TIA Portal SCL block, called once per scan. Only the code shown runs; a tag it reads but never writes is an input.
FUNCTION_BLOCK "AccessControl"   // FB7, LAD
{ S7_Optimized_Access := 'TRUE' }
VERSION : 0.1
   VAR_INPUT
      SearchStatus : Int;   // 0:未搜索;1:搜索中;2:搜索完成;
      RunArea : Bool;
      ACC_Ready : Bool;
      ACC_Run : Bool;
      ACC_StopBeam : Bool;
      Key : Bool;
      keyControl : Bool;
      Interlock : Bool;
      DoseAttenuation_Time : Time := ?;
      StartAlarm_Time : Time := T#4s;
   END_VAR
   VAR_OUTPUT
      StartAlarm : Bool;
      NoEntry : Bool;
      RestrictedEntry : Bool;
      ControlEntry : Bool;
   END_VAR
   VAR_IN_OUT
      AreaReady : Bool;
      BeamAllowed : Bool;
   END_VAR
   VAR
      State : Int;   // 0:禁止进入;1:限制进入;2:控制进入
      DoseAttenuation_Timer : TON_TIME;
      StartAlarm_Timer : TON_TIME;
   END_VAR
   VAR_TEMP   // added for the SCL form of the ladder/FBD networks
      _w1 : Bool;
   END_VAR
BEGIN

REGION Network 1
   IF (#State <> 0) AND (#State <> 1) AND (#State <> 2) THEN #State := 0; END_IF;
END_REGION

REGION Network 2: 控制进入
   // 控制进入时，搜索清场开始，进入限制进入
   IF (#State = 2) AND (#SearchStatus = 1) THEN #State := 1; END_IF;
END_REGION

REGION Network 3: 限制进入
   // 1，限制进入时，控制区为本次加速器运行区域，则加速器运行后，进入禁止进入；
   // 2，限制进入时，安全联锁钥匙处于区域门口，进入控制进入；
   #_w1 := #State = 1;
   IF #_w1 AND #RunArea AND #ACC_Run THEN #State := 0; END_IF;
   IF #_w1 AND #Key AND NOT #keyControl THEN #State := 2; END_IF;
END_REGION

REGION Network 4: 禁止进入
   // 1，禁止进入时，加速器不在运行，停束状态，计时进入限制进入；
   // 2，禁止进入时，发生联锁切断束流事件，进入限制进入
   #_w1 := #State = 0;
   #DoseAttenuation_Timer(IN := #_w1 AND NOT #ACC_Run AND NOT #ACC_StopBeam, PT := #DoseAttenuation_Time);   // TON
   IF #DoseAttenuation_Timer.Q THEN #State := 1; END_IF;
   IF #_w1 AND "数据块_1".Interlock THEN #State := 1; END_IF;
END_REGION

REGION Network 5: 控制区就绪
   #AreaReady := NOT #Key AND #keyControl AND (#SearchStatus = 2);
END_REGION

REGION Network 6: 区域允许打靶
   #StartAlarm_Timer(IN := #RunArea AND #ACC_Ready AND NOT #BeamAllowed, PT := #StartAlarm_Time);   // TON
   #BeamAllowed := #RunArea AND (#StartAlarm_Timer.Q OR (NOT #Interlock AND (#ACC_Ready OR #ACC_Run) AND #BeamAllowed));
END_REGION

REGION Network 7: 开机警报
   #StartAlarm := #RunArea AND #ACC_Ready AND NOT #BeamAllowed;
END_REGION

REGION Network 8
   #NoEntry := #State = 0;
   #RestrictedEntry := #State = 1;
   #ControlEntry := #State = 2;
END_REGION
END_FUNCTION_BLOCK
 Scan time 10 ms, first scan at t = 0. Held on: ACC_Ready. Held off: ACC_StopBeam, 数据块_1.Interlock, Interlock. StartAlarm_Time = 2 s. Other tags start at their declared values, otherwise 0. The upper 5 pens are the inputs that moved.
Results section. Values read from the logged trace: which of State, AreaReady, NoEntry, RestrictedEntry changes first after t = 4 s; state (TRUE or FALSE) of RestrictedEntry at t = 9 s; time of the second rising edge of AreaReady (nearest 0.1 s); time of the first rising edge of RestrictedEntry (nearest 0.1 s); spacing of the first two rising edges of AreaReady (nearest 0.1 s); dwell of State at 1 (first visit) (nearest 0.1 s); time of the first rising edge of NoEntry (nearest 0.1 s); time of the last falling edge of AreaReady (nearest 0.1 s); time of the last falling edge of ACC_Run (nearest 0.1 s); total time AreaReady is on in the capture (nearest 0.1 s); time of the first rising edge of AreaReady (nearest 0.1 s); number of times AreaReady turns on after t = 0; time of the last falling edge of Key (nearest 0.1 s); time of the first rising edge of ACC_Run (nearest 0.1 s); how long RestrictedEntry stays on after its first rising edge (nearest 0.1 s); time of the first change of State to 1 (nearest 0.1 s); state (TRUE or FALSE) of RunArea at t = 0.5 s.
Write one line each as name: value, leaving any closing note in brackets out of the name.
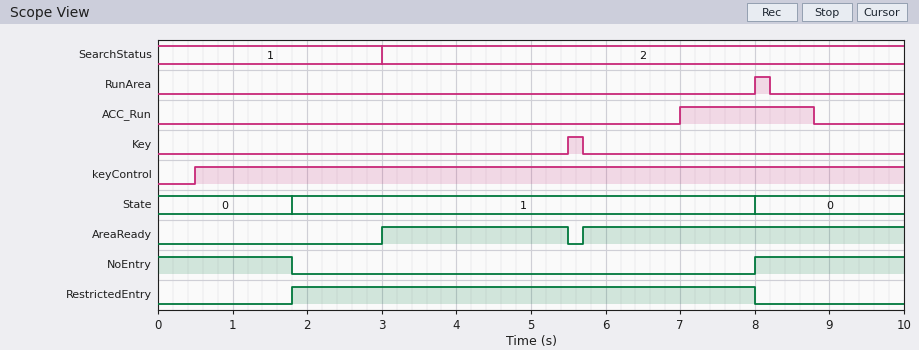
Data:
which of State, AreaReady, NoEntry, RestrictedEntry changes first after t = 4 s: AreaReady
state (TRUE or FALSE) of RestrictedEntry at t = 9 s: FALSE
time of the second rising edge of AreaReady: 5.7 s
time of the first rising edge of RestrictedEntry: 1.8 s
spacing of the first two rising edges of AreaReady: 2.7 s
dwell of State at 1 (first visit): 6.2 s
time of the first rising edge of NoEntry: 8.0 s
time of the last falling edge of AreaReady: 5.5 s
time of the last falling edge of ACC_Run: 8.8 s
total time AreaReady is on in the capture: 6.8 s
time of the first rising edge of AreaReady: 3.0 s
number of times AreaReady turns on after t = 0: 2
time of the last falling edge of Key: 5.7 s
time of the first rising edge of ACC_Run: 7.0 s
how long RestrictedEntry stays on after its first rising edge: 6.2 s
time of the first change of State to 1: 1.8 s
state (TRUE or FALSE) of RunArea at t = 0.5 s: FALSE
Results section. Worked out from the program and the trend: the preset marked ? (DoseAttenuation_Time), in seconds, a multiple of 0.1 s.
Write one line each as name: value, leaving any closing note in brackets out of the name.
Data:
the preset marked ? (DoseAttenuation_Time), in seconds, a multiple of 0.1 s: 1.8 s
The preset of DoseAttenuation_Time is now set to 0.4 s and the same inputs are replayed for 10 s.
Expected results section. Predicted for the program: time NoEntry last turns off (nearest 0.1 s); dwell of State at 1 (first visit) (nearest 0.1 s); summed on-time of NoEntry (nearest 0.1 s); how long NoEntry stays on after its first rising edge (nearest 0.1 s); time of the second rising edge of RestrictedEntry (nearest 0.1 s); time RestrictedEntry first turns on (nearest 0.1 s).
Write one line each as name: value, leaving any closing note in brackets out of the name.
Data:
time NoEntry last turns off: 9.2 s
dwell of State at 1 (first visit): 7.6 s
summed on-time of NoEntry: 1.6 s
how long NoEntry stays on after its first rising edge: 1.2 s
time of the second rising edge of RestrictedEntry: 9.2 s
time RestrictedEntry first turns on: 0.4 s
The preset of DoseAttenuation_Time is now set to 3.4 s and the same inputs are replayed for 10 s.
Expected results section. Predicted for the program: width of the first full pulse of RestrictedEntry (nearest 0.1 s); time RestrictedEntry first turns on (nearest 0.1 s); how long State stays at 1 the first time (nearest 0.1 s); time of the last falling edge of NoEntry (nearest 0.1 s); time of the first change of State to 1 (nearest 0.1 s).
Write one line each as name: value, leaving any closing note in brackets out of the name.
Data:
width of the first full pulse of RestrictedEntry: 4.6 s
time RestrictedEntry first turns on: 3.4 s
how long State stays at 1 the first time: 4.6 s
time of the last falling edge of NoEntry: 3.4 s
time of the first change of State to 1: 3.4 s
